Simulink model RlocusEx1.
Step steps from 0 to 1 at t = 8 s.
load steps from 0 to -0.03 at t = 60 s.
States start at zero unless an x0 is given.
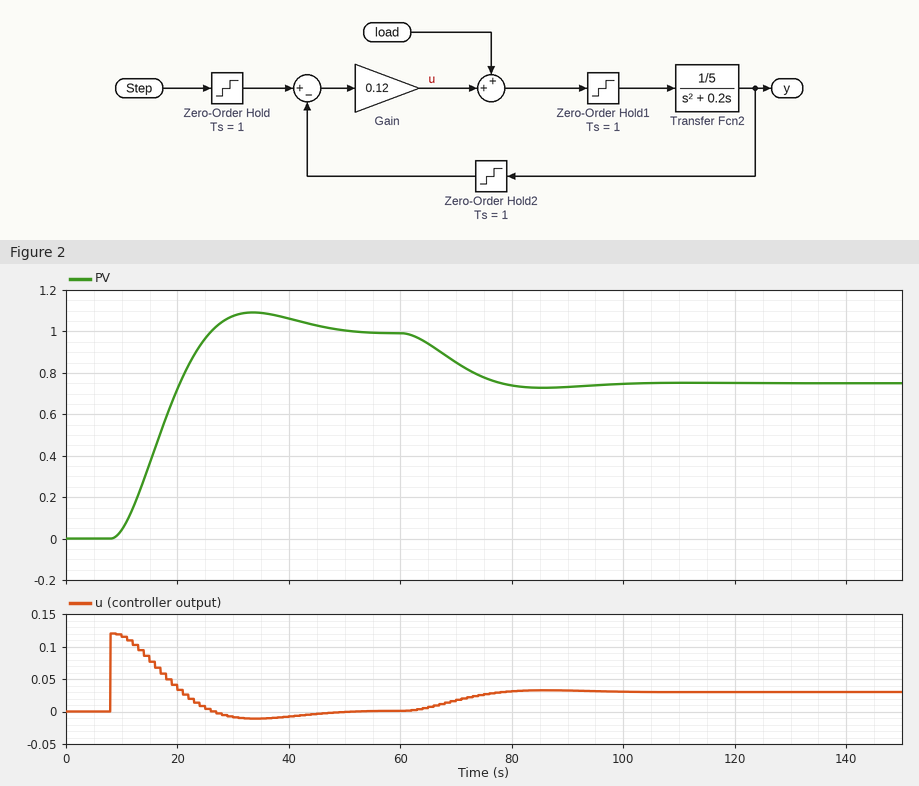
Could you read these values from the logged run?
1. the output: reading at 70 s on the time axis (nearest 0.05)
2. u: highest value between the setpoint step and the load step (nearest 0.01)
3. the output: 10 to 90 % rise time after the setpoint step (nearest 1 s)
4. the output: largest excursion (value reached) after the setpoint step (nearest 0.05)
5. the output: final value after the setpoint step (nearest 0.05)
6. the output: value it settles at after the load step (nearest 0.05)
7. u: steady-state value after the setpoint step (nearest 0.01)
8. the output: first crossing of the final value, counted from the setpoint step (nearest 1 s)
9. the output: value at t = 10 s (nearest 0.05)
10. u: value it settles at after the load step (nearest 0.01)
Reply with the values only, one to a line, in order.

0.85
0.12
12 s
1.10
1.00
0.75
0.00
18 s
0.05
0.03
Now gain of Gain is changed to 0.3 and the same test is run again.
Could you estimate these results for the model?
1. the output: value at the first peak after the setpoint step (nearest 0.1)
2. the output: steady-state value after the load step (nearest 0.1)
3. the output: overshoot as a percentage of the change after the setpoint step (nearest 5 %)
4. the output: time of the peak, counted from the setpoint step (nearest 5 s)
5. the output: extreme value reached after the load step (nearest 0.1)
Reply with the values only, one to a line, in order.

1.3
0.9
30 %
15 s
0.9
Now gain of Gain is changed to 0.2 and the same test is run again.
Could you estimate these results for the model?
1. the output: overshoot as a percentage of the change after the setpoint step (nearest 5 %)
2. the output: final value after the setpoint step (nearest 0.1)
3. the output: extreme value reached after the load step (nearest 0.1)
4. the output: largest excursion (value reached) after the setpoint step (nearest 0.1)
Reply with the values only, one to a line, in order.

20 %
1.0
0.8
1.2
